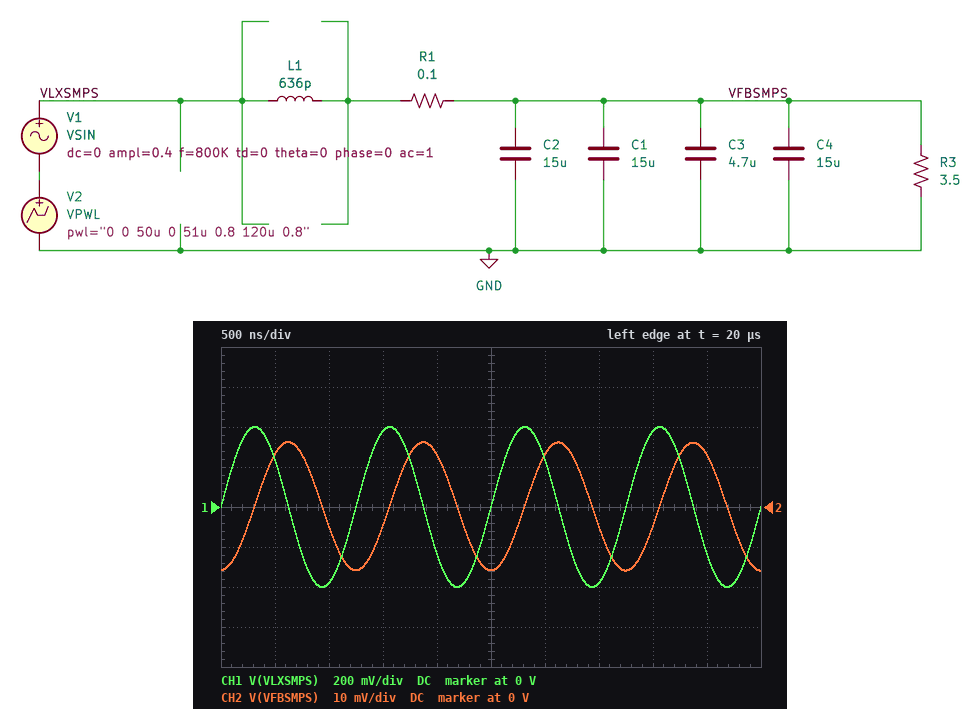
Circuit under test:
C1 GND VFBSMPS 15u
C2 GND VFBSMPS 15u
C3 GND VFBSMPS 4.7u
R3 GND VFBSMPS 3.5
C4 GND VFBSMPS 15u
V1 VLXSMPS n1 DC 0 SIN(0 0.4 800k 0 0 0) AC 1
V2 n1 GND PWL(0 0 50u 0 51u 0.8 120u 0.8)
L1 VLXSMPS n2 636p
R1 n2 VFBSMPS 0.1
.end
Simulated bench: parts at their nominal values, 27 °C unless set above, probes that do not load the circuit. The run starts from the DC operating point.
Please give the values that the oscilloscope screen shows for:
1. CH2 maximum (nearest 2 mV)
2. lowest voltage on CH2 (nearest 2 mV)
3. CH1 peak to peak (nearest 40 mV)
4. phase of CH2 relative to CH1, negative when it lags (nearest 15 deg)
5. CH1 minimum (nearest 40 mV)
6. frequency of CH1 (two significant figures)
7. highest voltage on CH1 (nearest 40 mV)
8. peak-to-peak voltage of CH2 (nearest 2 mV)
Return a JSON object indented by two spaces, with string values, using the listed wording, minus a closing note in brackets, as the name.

{
  "CH2 maximum": "16 mV",
  "lowest voltage on CH2": "-16 mV",
  "CH1 peak to peak": "800 mV",
  "phase of CH2 relative to CH1, negative when it lags": "-90 deg",
  "CH1 minimum": "-400 mV",
  "frequency of CH1": "800 kHz",
  "highest voltage on CH1": "400 mV",
  "peak-to-peak voltage of CH2": "32 mV"
}
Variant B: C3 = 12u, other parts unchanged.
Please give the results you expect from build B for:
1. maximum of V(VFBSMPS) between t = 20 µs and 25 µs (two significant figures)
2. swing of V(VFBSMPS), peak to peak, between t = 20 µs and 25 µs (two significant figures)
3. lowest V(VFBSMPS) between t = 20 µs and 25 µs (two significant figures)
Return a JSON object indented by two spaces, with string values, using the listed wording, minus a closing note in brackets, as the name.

{
  "maximum of V(VFBSMPS) between t = 20 µs and 25 µs": "14 mV",
  "swing of V(VFBSMPS), peak to peak, between t = 20 µs and 25 µs": "28 mV",
  "lowest V(VFBSMPS) between t = 20 µs and 25 µs": "-14 mV"
}
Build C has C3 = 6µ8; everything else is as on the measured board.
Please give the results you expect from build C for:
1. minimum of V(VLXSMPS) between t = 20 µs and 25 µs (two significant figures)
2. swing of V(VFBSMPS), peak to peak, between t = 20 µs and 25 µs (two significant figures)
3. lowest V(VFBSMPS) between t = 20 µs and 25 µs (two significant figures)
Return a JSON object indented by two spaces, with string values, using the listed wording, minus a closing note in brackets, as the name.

{
  "minimum of V(VLXSMPS) between t = 20 µs and 25 µs": "-400 mV",
  "swing of V(VFBSMPS), peak to peak, between t = 20 µs and 25 µs": "31 mV",
  "lowest V(VFBSMPS) between t = 20 µs and 25 µs": "-15 mV"
}
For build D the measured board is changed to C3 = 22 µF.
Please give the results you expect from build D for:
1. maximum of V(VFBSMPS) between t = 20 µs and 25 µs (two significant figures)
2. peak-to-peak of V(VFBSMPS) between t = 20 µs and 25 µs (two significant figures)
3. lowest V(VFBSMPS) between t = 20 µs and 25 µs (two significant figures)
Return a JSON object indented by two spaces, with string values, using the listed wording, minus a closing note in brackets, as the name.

{
  "maximum of V(VFBSMPS) between t = 20 µs and 25 µs": "12 mV",
  "peak-to-peak of V(VFBSMPS) between t = 20 µs and 25 µs": "24 mV",
  "lowest V(VFBSMPS) between t = 20 µs and 25 µs": "-12 mV"
}
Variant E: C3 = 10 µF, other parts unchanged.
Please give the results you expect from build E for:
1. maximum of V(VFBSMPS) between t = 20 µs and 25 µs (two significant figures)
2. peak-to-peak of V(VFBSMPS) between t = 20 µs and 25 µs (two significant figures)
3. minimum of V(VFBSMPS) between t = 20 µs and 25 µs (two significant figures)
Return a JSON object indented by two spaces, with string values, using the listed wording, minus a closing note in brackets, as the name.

{
  "maximum of V(VFBSMPS) between t = 20 µs and 25 µs": "15 mV",
  "peak-to-peak of V(VFBSMPS) between t = 20 µs and 25 µs": "29 mV",
  "minimum of V(VFBSMPS) between t = 20 µs and 25 µs": "-14 mV"
}
